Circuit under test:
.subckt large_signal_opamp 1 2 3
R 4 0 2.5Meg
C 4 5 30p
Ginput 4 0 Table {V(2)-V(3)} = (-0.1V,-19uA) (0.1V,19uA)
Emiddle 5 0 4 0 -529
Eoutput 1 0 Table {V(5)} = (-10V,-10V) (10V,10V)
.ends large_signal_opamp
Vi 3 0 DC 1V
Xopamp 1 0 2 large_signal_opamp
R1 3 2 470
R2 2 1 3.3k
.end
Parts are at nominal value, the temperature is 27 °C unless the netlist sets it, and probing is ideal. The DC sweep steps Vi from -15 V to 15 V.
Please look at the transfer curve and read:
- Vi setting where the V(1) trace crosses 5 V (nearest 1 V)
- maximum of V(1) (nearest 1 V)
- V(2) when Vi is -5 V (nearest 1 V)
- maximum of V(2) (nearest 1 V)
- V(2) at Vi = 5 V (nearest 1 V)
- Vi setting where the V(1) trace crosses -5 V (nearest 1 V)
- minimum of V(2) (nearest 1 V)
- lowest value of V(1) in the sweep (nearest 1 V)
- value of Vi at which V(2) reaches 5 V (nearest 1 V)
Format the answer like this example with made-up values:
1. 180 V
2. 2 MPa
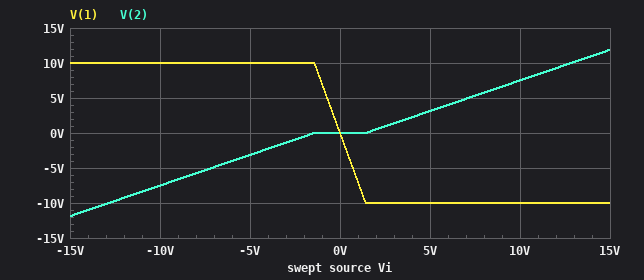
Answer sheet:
1. -1 V
2. 10 V
3. -3 V
4. 12 V
5. 3 V
6. 1 V
7. -12 V
8. -10 V
9. 7 V
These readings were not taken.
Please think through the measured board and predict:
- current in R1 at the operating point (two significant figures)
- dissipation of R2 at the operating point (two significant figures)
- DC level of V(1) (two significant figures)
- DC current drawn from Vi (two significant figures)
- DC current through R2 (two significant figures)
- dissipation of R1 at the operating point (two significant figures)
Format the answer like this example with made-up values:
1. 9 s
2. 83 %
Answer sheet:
1. 2.1 mA
2. 15 mW
3. -7.0 V
4. 2.1 mA
5. 2.1 mA
6. 2.1 mW
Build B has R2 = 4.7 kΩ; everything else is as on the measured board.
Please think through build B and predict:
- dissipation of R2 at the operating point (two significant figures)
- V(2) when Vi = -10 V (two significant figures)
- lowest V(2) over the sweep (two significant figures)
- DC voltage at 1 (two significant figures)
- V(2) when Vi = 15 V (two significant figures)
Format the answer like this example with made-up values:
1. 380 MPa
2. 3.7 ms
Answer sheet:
1. 21 mW
2. -8.2 V
3. -13 V
4. -10 V
5. 13 V
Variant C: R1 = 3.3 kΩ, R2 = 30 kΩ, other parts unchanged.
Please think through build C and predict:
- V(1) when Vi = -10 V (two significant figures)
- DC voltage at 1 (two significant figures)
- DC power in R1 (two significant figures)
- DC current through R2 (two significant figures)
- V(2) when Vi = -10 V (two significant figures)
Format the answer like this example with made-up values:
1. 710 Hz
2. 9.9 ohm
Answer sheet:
1. 10 V
2. -9.1 V
3. 300 µW
4. 300 µA
5. -8.0 V
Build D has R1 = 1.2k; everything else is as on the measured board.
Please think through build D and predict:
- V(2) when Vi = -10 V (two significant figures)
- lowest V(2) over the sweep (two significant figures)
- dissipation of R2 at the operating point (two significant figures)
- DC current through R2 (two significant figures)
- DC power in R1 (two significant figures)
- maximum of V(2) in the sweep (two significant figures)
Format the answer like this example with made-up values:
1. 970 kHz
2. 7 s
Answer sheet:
1. -4.7 V
2. -8.3 V
3. 2.3 mW
4. 830 µA
5. 830 µW
6. 8.3 V
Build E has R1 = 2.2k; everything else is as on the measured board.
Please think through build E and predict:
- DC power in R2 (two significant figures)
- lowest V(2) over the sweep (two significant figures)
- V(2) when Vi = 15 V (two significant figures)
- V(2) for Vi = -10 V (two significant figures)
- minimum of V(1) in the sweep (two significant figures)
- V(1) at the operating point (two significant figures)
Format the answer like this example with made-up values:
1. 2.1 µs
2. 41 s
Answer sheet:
1. 680 µW
2. -5.0 V
3. 5.0 V
4. -2.0 V
5. -10 V
6. -1.5 V
